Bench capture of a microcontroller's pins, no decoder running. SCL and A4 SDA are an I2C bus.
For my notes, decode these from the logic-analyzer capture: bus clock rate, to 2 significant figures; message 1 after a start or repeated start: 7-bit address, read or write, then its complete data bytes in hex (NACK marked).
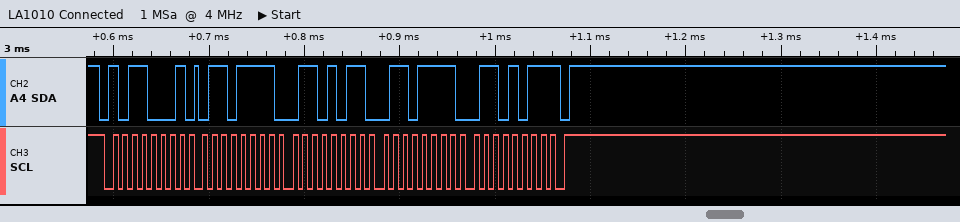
100 kHz
0x58 read: 6F 6B 6F 6B NACK
